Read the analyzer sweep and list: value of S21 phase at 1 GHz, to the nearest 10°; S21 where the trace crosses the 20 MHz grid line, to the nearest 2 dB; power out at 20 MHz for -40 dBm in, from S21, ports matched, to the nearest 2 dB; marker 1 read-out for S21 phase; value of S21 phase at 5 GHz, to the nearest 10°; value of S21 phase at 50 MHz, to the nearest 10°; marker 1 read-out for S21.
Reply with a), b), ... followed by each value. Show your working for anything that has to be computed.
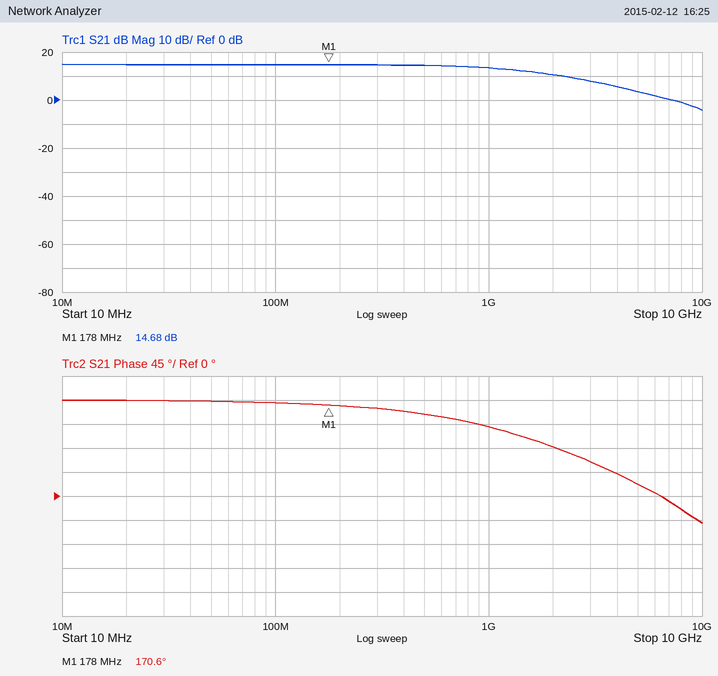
a) 130°
b) 14 dB
c) -40 dBm + (14 dB) = -26 dBm
d) 170.6°
e) 20°
f) 180°
g) 14.68 dB
